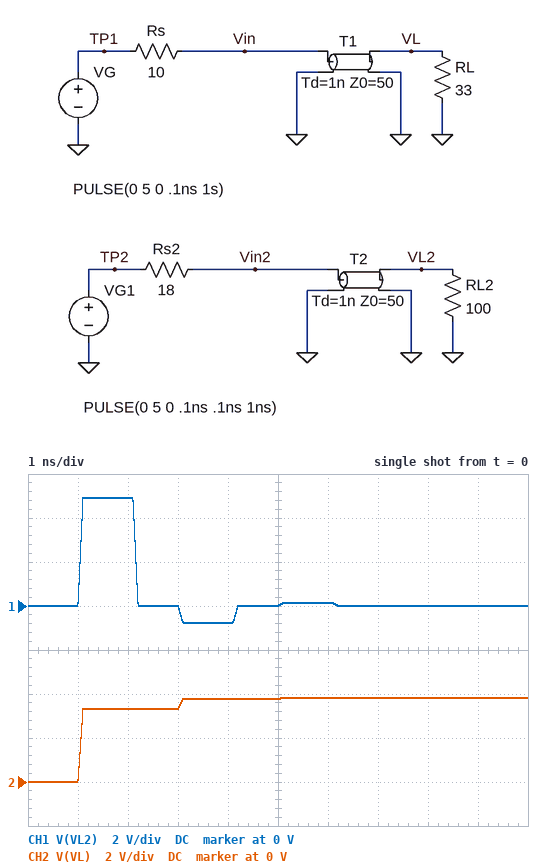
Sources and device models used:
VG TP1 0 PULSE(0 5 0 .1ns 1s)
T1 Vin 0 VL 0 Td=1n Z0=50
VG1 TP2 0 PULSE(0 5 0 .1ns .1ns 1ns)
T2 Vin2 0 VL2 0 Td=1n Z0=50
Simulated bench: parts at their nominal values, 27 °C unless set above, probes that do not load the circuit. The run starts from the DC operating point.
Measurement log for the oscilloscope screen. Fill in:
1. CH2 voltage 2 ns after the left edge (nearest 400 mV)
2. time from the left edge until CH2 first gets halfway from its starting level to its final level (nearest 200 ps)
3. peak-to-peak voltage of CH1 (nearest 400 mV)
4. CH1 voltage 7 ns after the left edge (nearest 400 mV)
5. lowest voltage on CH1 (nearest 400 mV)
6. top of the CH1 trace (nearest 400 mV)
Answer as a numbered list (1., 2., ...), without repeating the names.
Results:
1. 3.2 V
2. 1.0 ns
3. 5.6 V
4. 0 V
5. -800 mV
6. 4.8 V
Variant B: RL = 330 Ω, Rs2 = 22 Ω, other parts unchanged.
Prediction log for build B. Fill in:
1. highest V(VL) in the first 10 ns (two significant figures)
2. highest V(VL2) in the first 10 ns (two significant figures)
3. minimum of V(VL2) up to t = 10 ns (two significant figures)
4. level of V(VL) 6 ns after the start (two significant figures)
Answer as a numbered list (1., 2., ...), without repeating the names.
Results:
1. 7.2 V
2. 4.6 V
3. -600 mV
4. 5.4 V
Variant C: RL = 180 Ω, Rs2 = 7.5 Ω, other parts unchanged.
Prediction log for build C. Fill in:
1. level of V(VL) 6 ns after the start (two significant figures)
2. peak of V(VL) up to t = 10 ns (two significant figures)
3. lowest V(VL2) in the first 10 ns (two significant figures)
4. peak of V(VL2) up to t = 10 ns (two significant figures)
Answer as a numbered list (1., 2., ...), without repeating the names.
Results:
1. 5.0 V
2. 6.5 V
3. -1.4 V
4. 5.8 V
